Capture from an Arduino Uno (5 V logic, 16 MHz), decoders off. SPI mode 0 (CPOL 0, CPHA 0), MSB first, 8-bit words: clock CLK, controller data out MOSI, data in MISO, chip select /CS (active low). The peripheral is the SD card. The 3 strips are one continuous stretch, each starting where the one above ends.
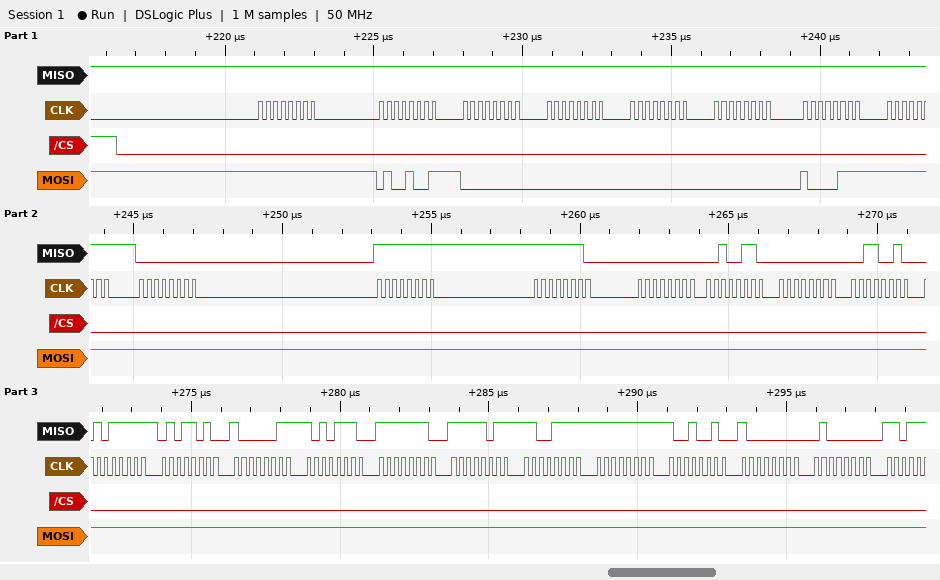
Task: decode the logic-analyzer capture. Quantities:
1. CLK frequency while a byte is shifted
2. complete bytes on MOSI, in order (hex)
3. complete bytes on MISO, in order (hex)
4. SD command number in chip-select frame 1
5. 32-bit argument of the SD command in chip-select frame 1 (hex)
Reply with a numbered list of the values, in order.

1. 4 MHz
2. FF 49 00 00 00 00 87 FF FF FF FF FF FF FF FF FF FF FF FF FF FF FF FF FF FF FF
3. FF FF FF FF FF FF FF FF 00 FF FE 00 26 00 32 5F 5A 83 AE FE FB CF FF 92 80 40
4. CMD9
5. 0x00000000
